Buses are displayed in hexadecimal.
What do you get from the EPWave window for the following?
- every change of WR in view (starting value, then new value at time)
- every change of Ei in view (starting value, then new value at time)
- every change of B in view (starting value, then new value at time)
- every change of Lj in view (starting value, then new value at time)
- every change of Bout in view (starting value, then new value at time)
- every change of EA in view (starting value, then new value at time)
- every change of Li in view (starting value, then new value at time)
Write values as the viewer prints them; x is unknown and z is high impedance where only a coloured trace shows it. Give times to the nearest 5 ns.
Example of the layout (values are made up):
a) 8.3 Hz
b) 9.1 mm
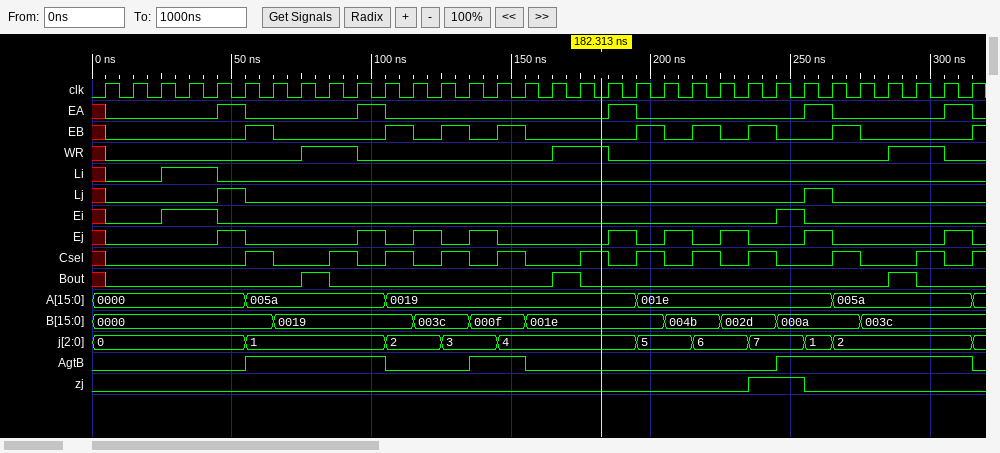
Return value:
a) x, 0 at 5 ns, 1 at 75 ns, 0 at 95 ns, 1 at 165 ns, 0 at 185 ns, 1 at 285 ns, 0 at 305 ns
b) x, 0 at 5 ns, 1 at 25 ns, 0 at 45 ns, 1 at 245 ns, 0 at 255 ns
c) 0000, 0019 at 65 ns, 003c at 115 ns, 000f at 135 ns, 001e at 155 ns, 004b at 205 ns, 002d at 225 ns, 000a at 245 ns, 003c at 275 ns
d) x, 0 at 5 ns, 1 at 45 ns, 0 at 55 ns, 1 at 255 ns, 0 at 265 ns
e) x, 0 at 5 ns, 1 at 75 ns, 0 at 85 ns, 1 at 165 ns, 0 at 175 ns, 1 at 285 ns, 0 at 295 ns
f) x, 0 at 5 ns, 1 at 45 ns, 0 at 55 ns, 1 at 95 ns, 0 at 105 ns, 1 at 185 ns, 0 at 195 ns, 1 at 255 ns, 0 at 265 ns, 1 at 305 ns, 0 at 315 ns
g) x, 0 at 5 ns, 1 at 25 ns, 0 at 45 ns
